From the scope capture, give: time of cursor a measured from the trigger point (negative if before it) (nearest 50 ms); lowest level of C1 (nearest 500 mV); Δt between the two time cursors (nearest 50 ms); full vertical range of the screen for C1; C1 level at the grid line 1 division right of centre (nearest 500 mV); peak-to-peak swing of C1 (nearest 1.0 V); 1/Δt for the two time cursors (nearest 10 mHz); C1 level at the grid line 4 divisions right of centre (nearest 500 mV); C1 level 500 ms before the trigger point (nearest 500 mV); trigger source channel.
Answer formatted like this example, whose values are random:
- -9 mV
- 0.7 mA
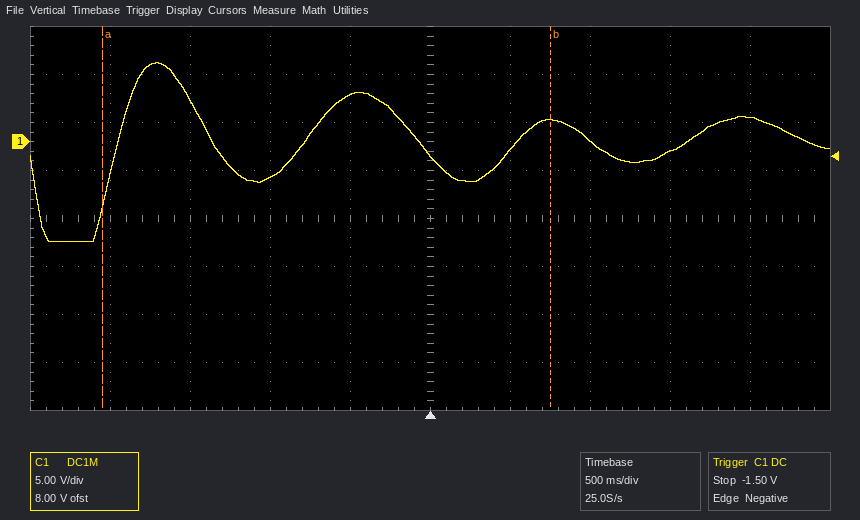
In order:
- -2.05 s
- -10.5 V
- 2.80 s
- 40 V
- -1.0 V
- 19.0 V
- 360 mHz
- 2.5 V
- 5.0 V
- C1
